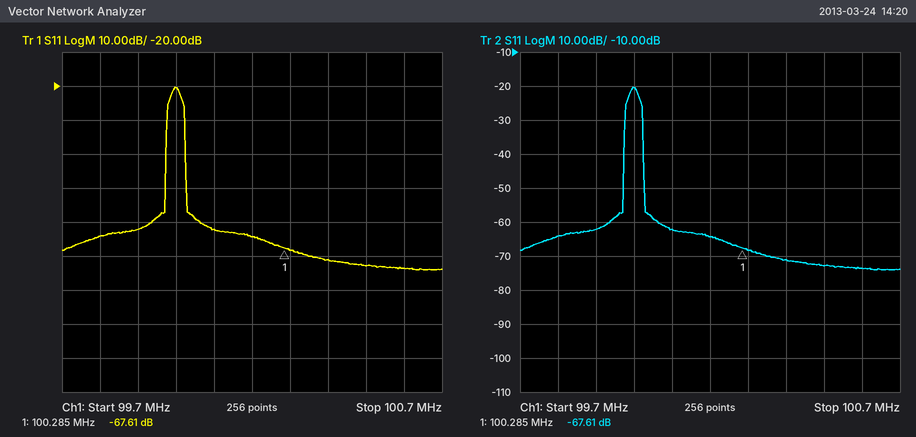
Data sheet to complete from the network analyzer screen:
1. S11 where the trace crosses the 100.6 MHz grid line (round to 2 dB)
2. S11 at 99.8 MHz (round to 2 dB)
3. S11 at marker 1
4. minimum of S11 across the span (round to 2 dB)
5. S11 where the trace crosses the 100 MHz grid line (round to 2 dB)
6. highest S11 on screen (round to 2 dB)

-74 dB
-64 dB
-67.61 dB
-74 dB
-20 dB
-20 dB
